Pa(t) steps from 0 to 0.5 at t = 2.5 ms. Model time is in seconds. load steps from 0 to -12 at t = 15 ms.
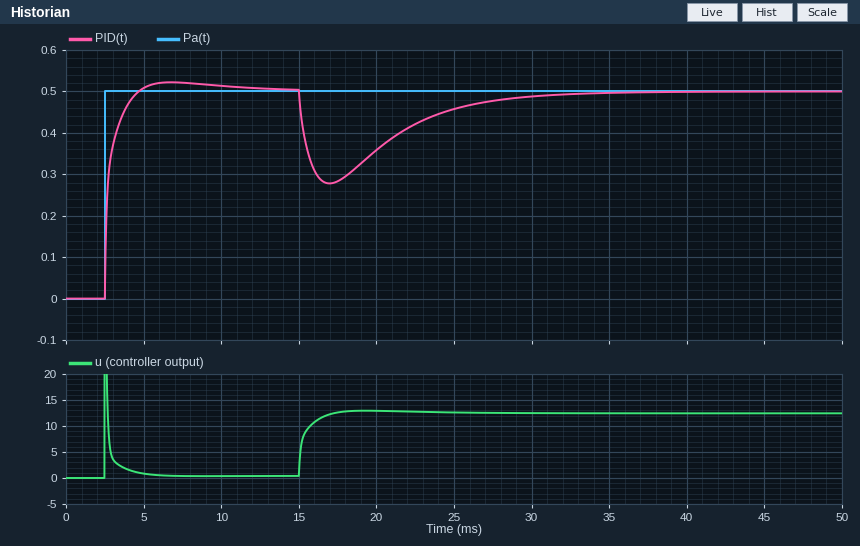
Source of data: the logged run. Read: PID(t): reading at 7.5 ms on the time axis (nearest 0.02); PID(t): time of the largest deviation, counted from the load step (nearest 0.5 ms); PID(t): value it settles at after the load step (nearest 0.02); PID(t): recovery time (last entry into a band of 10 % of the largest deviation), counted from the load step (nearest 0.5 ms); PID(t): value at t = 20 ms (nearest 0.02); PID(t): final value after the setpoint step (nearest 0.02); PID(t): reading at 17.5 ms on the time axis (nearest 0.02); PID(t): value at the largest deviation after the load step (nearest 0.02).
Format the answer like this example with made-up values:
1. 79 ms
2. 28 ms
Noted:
1. 0.52
2. 2.0 ms
3. 0.50
4. 12.5 ms
5. 0.36
6. 0.50
7. 0.28
8. 0.28
